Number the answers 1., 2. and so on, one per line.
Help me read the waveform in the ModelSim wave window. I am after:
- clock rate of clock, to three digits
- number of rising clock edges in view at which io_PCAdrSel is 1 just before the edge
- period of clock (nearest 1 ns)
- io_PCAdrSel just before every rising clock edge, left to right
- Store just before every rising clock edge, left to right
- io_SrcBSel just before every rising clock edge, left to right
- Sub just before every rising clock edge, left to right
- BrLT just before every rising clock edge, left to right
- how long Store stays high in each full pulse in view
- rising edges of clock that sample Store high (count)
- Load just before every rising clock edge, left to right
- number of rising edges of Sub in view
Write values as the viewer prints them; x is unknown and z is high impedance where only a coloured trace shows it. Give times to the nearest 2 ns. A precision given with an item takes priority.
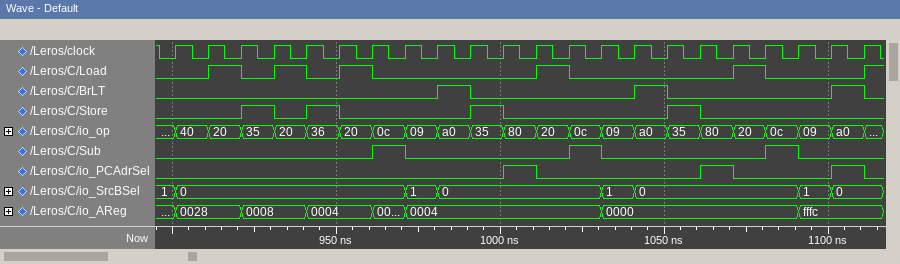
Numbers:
1. 100 MHz
2. 3
3. 10 ns
4. 0 0 0 0 0 0 0 0 0 0 0 1 0 0 0 0 0 1 0 0 0 1
5. 0 0 0 1 0 1 0 0 0 0 1 0 0 0 0 0 1 0 0 0 0 0
6. 1, 0, 0, 0, 0, 0, 0, 0, 1, 0, 0, 0, 0, 0, 1, 0, 0, 0, 0, 0, 1, 0
7. 0 0 0 0 0 0 0 1 0 0 0 0 0 1 0 0 0 0 0 1 0 0
8. 0 0 0 0 0 0 0 0 0 1 0 0 0 0 0 1 0 0 0 0 0 1
9. 10 ns, 10 ns, 10 ns, 10 ns
10. 4
11. 0 0 1 0 1 0 1 0 0 0 0 0 1 0 0 0 0 0 1 0 0 0
12. 3
